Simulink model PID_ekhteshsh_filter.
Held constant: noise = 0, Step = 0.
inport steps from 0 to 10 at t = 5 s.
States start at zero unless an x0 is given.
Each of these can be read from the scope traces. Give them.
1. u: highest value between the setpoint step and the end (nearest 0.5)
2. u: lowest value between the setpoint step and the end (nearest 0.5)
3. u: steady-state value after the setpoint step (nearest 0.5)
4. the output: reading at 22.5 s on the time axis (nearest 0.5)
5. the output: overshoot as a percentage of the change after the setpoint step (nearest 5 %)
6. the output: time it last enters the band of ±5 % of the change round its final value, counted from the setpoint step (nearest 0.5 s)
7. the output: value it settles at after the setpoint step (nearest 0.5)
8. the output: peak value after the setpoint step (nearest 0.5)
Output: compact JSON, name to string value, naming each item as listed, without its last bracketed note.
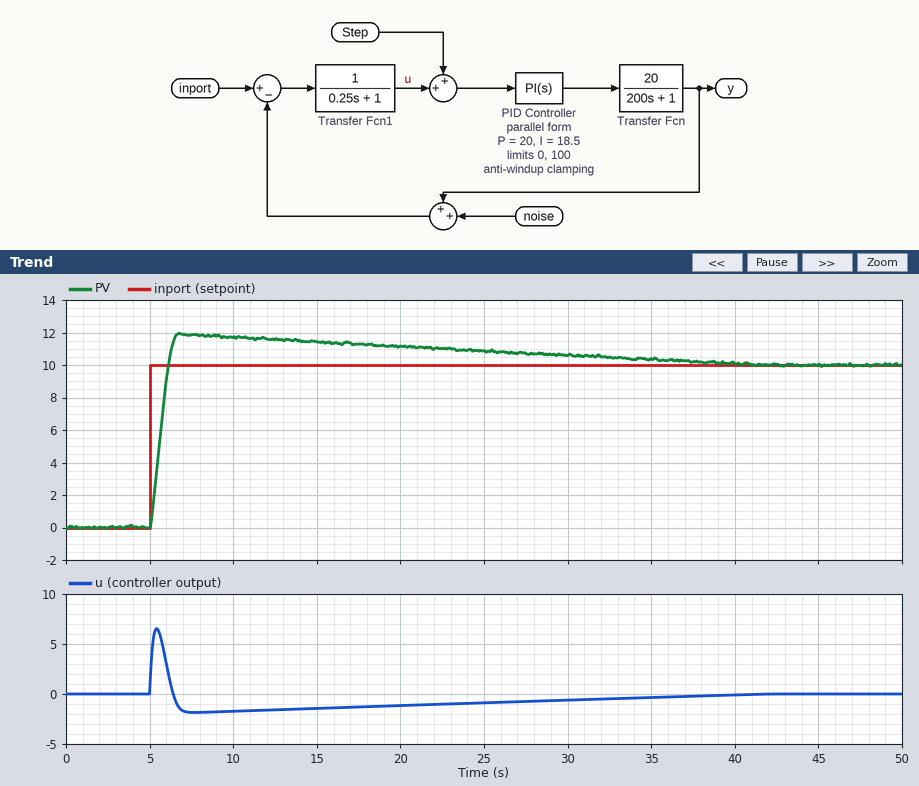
{"u: highest value between the setpoint step and the end": "6.5", "u: lowest value between the setpoint step and the end": "-2.0", "u: steady-state value after the setpoint step": "0.0", "the output: reading at 22.5 s on the time axis": "11.0", "the output: overshoot as a percentage of the change after the setpoint step": "20 %", "the output: time it last enters the band of ±5 % of the change round its final value, counted from the setpoint step": "27.0 s", "the output: value it settles at after the setpoint step": "10.0", "the output: peak value after the setpoint step": "12.0"}
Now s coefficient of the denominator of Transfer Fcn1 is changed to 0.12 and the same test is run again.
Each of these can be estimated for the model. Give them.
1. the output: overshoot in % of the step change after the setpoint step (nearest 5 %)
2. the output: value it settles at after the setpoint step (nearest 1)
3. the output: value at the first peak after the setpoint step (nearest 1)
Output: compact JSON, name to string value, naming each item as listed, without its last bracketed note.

{"the output: overshoot in % of the step change after the setpoint step": "10 %", "the output: value it settles at after the setpoint step": "10", "the output: value at the first peak after the setpoint step": "11"}
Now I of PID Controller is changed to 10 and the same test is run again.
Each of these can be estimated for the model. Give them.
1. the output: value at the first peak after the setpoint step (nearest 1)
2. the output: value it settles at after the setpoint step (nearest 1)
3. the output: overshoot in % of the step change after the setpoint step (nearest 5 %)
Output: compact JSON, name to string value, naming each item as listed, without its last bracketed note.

{"the output: value at the first peak after the setpoint step": "11", "the output: value it settles at after the setpoint step": "10", "the output: overshoot in % of the step change after the setpoint step": "15 %"}
